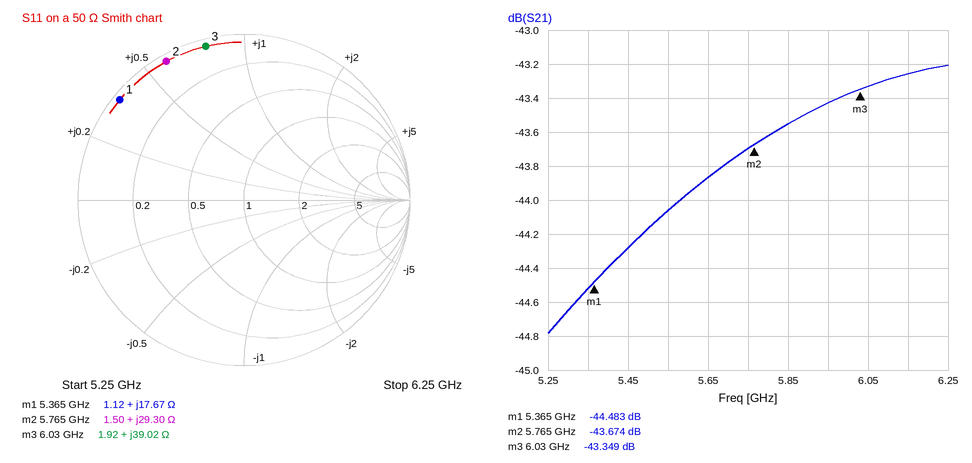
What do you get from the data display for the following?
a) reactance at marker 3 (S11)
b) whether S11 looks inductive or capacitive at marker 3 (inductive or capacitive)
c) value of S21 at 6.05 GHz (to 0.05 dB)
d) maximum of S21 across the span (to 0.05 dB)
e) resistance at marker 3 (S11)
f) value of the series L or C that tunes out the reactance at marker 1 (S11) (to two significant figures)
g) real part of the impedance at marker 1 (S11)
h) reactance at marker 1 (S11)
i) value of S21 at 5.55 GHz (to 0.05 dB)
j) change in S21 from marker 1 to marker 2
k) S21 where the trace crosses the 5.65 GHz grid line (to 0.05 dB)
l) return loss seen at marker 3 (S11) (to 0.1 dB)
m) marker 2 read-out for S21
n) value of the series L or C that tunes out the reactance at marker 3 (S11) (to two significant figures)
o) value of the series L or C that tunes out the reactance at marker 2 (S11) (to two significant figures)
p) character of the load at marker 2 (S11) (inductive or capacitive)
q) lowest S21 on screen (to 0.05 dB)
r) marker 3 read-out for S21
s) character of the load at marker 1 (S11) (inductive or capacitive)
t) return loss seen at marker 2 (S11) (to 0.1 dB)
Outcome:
+39.02 Ω
inductive
-43.35 dB
-43.20 dB
1.92 Ω
1.7 pF
1.12 Ω
+17.67 Ω
-44.05 dB
0.809 dB
-43.85 dB
0.4 dB
-43.674 dB
680 fF
940 fF
inductive
-44.80 dB
-43.349 dB
inductive
0.4 dB
